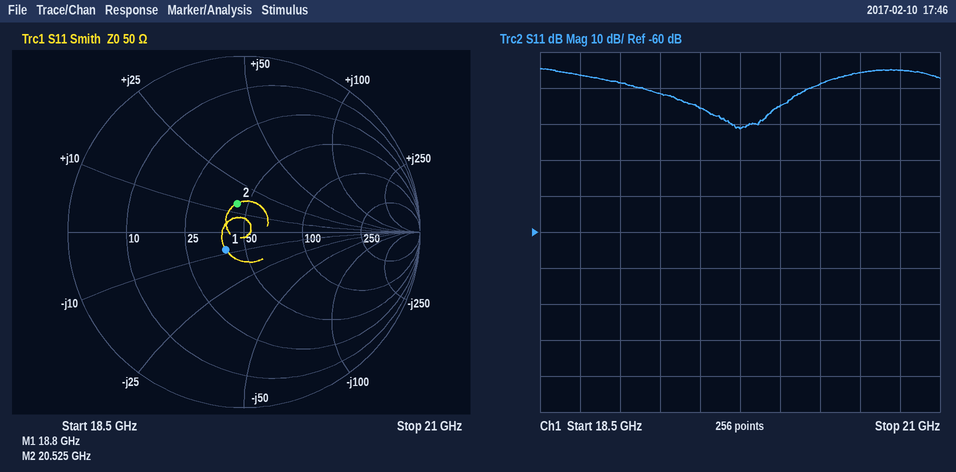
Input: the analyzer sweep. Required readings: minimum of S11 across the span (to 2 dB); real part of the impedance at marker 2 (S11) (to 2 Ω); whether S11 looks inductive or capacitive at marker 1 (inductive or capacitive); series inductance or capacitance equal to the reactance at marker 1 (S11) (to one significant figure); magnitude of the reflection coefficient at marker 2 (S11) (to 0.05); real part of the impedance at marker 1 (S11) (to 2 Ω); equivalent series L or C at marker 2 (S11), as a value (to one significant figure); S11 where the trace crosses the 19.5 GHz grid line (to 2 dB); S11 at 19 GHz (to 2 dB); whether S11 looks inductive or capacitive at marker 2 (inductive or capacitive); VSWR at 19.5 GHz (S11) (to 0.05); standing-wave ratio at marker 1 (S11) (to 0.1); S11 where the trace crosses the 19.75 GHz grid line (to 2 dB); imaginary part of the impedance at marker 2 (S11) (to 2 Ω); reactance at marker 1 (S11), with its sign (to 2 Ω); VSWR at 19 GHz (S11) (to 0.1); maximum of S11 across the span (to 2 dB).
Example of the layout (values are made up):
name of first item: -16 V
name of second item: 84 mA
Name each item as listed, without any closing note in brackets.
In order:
minimum of S11 across the span: -32 dB
real part of the impedance at marker 2 (S11): 44 Ω
whether S11 looks inductive or capacitive at marker 1: capacitive
series inductance or capacitance equal to the reactance at marker 1 (S11): 1 pF
magnitude of the reflection coefficient at marker 2 (S11): 0.15
real part of the impedance at marker 1 (S11): 40 Ω
equivalent series L or C at marker 2 (S11), as a value: 100 pH
S11 where the trace crosses the 19.5 GHz grid line: -26 dB
S11 at 19 GHz: -18 dB
whether S11 looks inductive or capacitive at marker 2: inductive
VSWR at 19.5 GHz (S11): 1.10
standing-wave ratio at marker 1 (S11): 1.3
S11 where the trace crosses the 19.75 GHz grid line: -32 dB
imaginary part of the impedance at marker 2 (S11): +14 Ω
reactance at marker 1 (S11), with its sign: -8 Ω
VSWR at 19 GHz (S11): 1.3
maximum of S11 across the span: -14 dB
